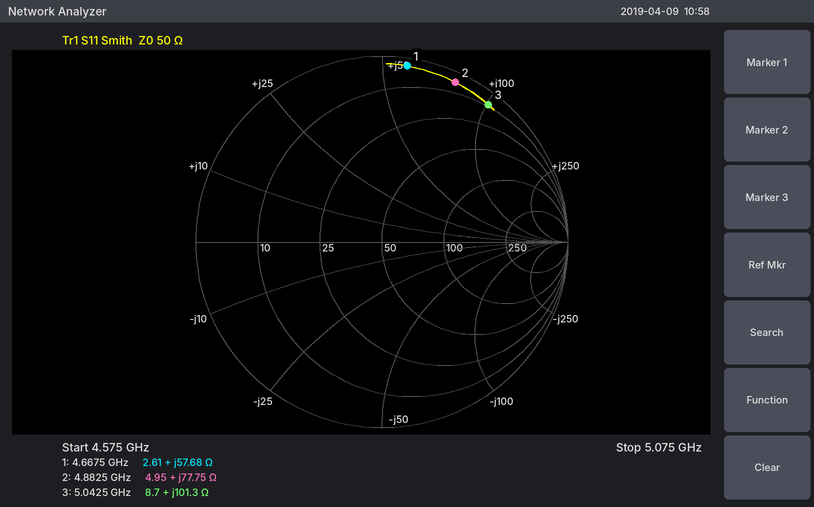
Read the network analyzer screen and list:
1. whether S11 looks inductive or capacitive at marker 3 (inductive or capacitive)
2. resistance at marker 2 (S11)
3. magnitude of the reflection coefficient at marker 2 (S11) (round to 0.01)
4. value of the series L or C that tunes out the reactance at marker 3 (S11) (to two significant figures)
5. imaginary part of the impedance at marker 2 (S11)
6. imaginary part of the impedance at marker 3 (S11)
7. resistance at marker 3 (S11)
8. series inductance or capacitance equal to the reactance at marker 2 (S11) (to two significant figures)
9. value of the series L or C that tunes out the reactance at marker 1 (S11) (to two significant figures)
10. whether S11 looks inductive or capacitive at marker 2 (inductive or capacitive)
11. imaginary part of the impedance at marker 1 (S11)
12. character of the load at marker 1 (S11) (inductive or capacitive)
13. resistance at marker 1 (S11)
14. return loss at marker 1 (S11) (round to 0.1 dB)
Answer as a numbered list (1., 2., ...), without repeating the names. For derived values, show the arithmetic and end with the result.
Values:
1. inductive
2. 4.95 Ω
3. 0.94
4. C = 1/(2π × 5.0425 GHz × 101.3 Ω) ≈ 312 fF, so 310 fF to two significant figures
5. +77.75 Ω
6. +101.3 Ω
7. 8.7 Ω
8. L = 77.75 Ω/(2π × 4.8825 GHz) ≈ 2.5 nH
9. C = 1/(2π × 4.6675 GHz × 57.68 Ω) ≈ 591 fF, so 590 fF to two significant figures
10. inductive
11. +57.68 Ω
12. inductive
13. 2.61 Ω
14. 0.4 dB
